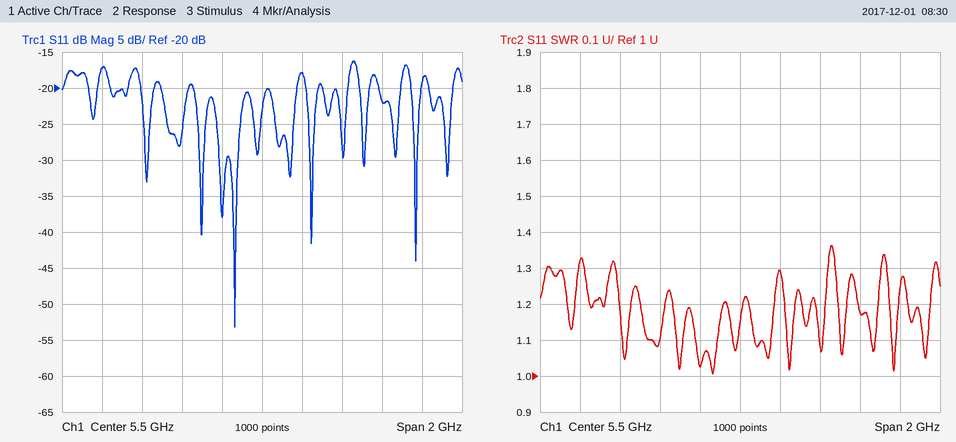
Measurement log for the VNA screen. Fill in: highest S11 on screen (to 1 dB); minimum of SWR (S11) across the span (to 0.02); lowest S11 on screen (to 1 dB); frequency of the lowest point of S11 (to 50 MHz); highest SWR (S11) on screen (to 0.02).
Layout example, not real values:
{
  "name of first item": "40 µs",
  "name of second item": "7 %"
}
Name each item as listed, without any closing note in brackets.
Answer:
{
  "highest S11 on screen": "-16 dB",
  "minimum of SWR (S11) across the span": "1.00",
  "lowest S11 on screen": "-53 dB",
  "frequency of the lowest point of S11": "5.35 GHz",
  "highest SWR (S11) on screen": "1.36"
}
